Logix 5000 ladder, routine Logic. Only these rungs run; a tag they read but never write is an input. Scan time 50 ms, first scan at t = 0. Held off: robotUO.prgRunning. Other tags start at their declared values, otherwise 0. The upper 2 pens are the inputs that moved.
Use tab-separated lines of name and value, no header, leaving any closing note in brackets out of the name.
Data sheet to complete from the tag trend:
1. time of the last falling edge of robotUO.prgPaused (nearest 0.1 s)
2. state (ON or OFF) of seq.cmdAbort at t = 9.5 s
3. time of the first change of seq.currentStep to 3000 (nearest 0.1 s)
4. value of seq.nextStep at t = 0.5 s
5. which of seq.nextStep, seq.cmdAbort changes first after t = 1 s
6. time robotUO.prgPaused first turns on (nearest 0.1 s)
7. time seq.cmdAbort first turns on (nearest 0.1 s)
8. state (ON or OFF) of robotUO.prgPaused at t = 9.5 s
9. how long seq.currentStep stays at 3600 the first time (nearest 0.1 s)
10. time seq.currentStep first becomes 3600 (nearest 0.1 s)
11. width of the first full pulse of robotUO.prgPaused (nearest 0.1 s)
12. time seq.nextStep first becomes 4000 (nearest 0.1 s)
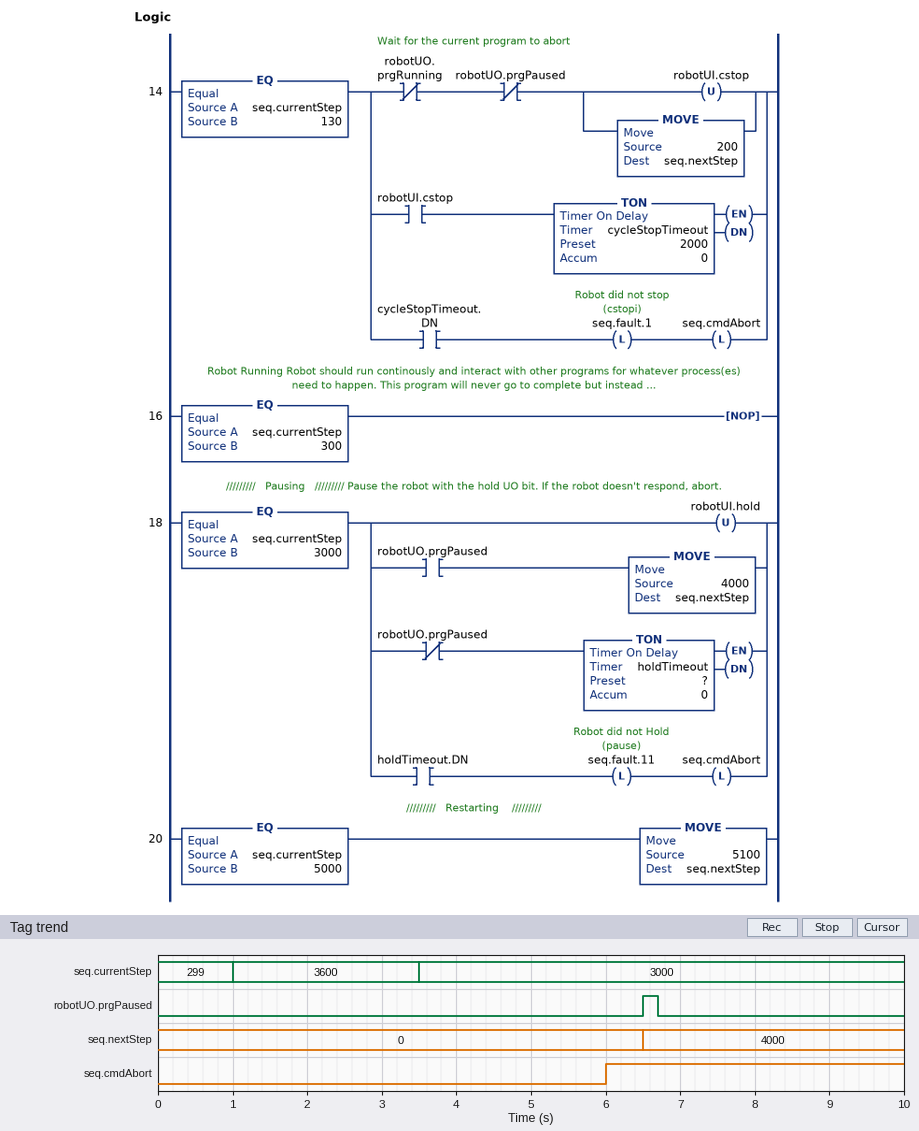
time of the last falling edge of robotUO.prgPaused	6.7 s
state (ON or OFF) of seq.cmdAbort at t = 9.5 s	ON
time of the first change of seq.currentStep to 3000	3.5 s
value of seq.nextStep at t = 0.5 s	0
which of seq.nextStep, seq.cmdAbort changes first after t = 1 s	seq.cmdAbort
time robotUO.prgPaused first turns on	6.5 s
time seq.cmdAbort first turns on	6.0 s
state (ON or OFF) of robotUO.prgPaused at t = 9.5 s	OFF
how long seq.currentStep stays at 3600 the first time	2.5 s
time seq.currentStep first becomes 3600	1.0 s
width of the first full pulse of robotUO.prgPaused	0.2 s
time seq.nextStep first becomes 4000	6.5 s
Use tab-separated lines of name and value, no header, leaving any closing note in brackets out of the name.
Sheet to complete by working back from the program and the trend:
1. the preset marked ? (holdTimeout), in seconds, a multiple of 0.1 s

the preset marked ? (holdTimeout), in seconds, a multiple of 0.1 s	2.5 s
